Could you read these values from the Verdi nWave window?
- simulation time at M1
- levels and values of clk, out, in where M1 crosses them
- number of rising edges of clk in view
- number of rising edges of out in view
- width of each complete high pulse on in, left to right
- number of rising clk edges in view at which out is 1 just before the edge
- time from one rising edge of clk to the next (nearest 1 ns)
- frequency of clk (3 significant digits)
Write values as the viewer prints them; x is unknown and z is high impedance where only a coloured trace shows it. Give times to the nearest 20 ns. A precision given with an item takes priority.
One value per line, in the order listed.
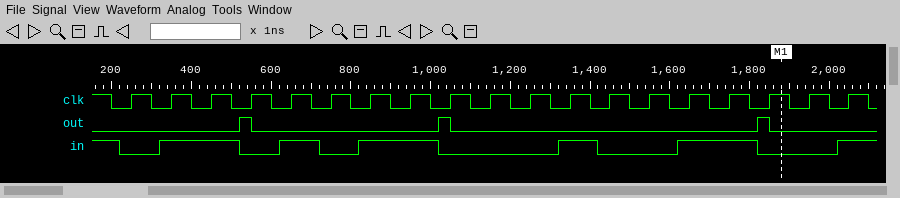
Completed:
1880 ns
clk=1, out=0, in=0
19
3
200 ns, 100 ns, 200 ns, 100 ns, 200 ns
3
100 ns
10.0 MHz
